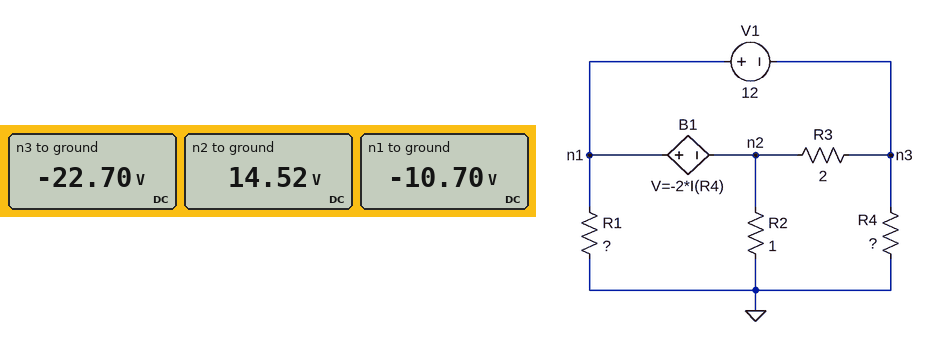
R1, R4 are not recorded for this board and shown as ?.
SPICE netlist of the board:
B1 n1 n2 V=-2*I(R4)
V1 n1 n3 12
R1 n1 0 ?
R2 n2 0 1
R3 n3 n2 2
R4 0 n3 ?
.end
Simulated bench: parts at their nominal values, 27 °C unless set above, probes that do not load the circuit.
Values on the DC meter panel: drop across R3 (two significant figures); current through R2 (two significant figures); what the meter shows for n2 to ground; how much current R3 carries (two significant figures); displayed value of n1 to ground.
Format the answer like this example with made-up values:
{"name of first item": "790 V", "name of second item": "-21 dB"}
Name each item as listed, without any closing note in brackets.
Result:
{"drop across R3": "37 V", "current through R2": "15 A", "what the meter shows for n2 to ground": "14.52 V", "how much current R3 carries": "19 A", "displayed value of n1 to ground": "-10.70 V"}
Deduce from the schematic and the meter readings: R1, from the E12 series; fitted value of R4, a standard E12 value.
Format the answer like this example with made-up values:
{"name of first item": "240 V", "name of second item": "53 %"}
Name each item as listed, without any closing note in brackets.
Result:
{"R1, from the E12 series": "5.6 Ω", "fitted value of R4, a standard E12 value": "1.8 Ω"}
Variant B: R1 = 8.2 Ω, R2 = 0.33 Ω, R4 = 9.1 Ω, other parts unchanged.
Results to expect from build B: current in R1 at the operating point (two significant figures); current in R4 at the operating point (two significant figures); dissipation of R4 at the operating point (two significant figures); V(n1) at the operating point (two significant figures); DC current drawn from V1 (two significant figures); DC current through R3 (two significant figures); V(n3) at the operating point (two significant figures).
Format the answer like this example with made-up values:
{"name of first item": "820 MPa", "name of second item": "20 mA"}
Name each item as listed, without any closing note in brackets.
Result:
{"current in R1 at the operating point": "310 mA", "current in R4 at the operating point": "1.6 A", "dissipation of R4 at the operating point": "23 W", "V(n1) at the operating point": "-2.6 V", "DC current drawn from V1": "9.2 A", "DC current through R3": "7.6 A", "V(n3) at the operating point": "-15 V"}
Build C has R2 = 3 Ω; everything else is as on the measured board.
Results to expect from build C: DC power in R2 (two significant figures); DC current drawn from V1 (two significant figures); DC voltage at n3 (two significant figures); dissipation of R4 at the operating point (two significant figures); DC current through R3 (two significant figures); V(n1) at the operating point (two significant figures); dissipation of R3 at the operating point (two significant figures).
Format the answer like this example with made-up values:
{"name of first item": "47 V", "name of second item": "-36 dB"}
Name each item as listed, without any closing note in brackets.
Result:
{"DC power in R2": "56 W", "DC current drawn from V1": "16 A", "DC voltage at n3": "-8.8 V", "dissipation of R4 at the operating point": "43 W", "DC current through R3": "11 A", "V(n1) at the operating point": "3.2 V", "dissipation of R3 at the operating point": "240 W"}
